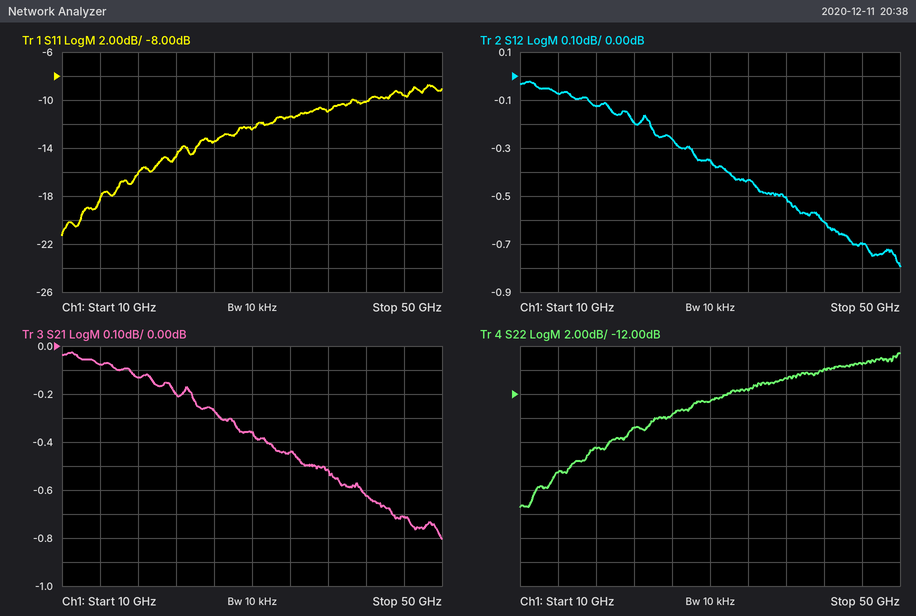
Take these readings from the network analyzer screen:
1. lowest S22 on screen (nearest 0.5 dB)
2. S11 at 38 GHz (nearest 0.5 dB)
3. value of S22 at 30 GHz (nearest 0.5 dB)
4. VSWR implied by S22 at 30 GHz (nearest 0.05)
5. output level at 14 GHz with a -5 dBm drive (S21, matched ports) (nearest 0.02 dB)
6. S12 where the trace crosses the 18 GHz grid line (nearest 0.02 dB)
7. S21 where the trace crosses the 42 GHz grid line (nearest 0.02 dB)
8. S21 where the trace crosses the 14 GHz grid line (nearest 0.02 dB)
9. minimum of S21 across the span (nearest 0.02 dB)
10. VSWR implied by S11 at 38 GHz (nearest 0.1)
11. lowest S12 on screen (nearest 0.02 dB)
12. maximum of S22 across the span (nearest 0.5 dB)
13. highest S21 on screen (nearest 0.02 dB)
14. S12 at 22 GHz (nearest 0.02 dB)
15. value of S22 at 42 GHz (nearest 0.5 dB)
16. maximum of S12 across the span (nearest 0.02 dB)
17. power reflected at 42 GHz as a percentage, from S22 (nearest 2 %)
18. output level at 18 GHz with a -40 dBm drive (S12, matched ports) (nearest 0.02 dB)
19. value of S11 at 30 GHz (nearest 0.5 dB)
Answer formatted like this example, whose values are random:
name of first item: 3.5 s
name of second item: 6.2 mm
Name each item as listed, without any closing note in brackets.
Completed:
lowest S22 on screen: -21.5 dB
S11 at 38 GHz: -11.0 dB
value of S22 at 30 GHz: -12.5 dB
VSWR implied by S22 at 30 GHz: 1.60
output level at 14 GHz with a -5 dBm drive (S21, matched ports): -5.08 dBm
S12 where the trace crosses the 18 GHz grid line: -0.12 dB
S21 where the trace crosses the 42 GHz grid line: -0.62 dB
S21 where the trace crosses the 14 GHz grid line: -0.08 dB
minimum of S21 across the span: -0.80 dB
VSWR implied by S11 at 38 GHz: 1.8
lowest S12 on screen: -0.80 dB
maximum of S22 across the span: -8.5 dB
highest S21 on screen: -0.02 dB
S12 at 22 GHz: -0.20 dB
value of S22 at 42 GHz: -10.0 dB
maximum of S12 across the span: -0.02 dB
power reflected at 42 GHz as a percentage, from S22: 10 %
output level at 18 GHz with a -40 dBm drive (S12, matched ports): -40.12 dBm
value of S11 at 30 GHz: -12.5 dB
